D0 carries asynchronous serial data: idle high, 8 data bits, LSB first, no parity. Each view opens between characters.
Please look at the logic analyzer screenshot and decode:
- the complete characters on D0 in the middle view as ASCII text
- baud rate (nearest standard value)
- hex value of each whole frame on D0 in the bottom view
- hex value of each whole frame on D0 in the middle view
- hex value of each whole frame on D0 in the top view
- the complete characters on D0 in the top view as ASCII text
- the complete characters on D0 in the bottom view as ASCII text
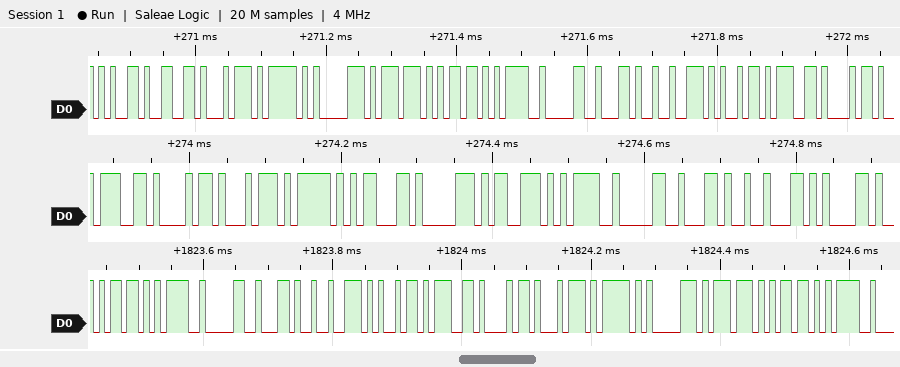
"ght_cps=0,ba"
115200 baud
6D, 3D, 30, 2C, 72, 69, 67, 68, 74, 5F, 70, 77, 6D, 3D
67, 68, 74, 5F, 63, 70, 73, 3D, 30, 2C, 62, 61
65, 66, 74, 5F, 70, 77, 6D, 3D, 30, 2C, 72, 69, 67, 68
"eft_pwm=0,righ"
"m=0,right_pwm="
